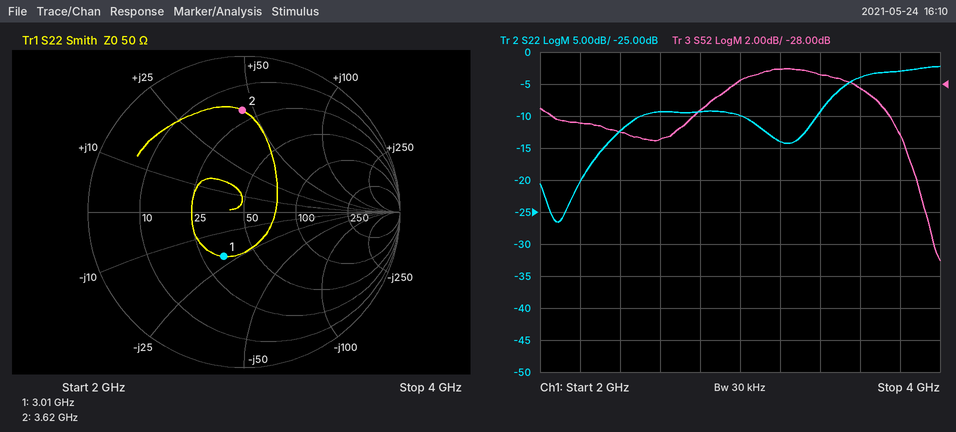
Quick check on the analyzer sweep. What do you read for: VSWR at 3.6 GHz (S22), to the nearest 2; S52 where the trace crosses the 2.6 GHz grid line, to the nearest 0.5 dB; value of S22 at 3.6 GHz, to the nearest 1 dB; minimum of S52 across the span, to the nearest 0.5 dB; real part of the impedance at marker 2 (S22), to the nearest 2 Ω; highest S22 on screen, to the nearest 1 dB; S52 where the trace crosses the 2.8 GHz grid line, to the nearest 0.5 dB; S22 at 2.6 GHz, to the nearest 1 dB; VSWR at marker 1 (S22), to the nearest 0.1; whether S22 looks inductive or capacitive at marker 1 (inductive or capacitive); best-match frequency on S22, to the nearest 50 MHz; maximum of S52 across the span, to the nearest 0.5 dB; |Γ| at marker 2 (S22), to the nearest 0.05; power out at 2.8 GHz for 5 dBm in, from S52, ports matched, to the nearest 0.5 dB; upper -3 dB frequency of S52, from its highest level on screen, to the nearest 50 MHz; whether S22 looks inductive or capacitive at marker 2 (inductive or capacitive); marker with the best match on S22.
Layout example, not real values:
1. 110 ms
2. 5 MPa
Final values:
1. 4
2. -31.5 dB
3. -4 dB
4. -39.0 dB
5. 20 Ω
6. -2 dB
7. -29.5 dB
8. -9 dB
9. 1.9
10. capacitive
11. 2.10 GHz
12. -27.0 dB
13. 0.65
14. -24.5 dBm
15. 3.75 GHz
16. inductive
17. marker 1
